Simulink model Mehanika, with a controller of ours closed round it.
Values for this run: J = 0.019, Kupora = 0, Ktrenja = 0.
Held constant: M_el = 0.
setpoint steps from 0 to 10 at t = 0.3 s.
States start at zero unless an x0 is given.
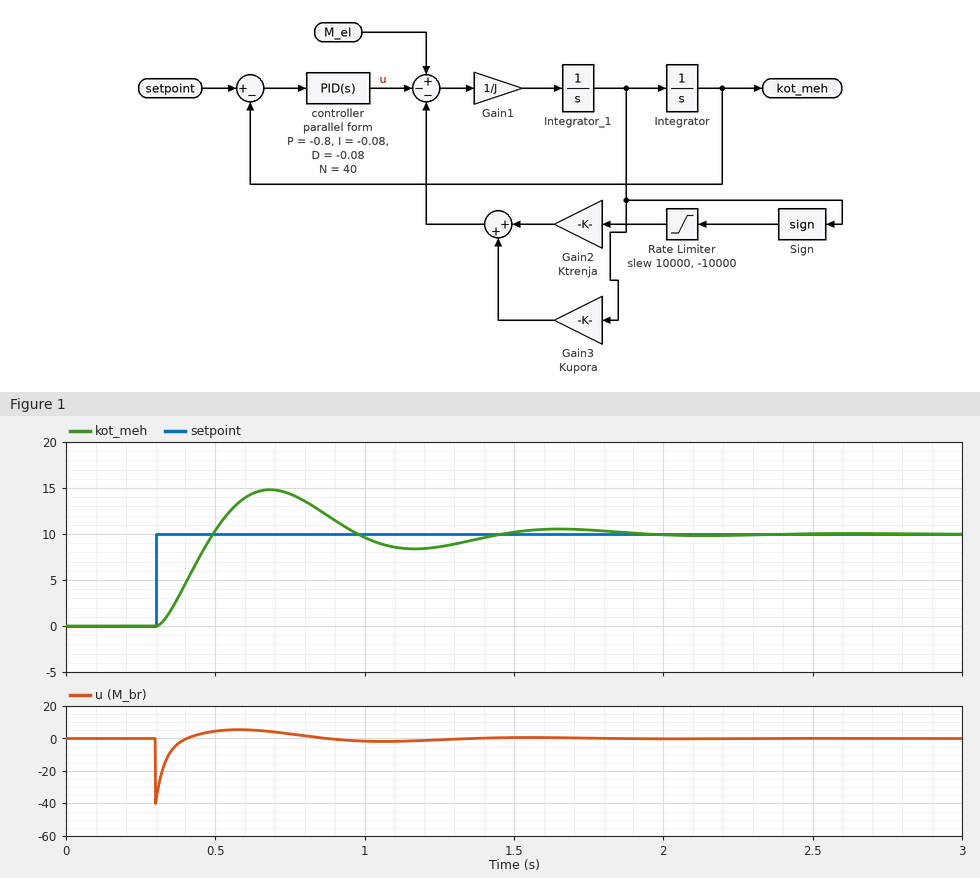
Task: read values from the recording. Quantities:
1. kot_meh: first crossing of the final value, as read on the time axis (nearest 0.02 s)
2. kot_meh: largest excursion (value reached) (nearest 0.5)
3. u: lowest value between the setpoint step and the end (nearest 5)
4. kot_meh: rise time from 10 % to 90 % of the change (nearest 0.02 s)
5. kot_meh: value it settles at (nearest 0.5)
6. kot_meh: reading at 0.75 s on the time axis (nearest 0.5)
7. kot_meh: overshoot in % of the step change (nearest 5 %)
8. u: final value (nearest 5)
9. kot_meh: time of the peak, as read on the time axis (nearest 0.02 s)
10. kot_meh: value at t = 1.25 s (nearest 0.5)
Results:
0.50 s
15.0
-40
0.14 s
10.0
14.5
50 %
0
0.68 s
8.5
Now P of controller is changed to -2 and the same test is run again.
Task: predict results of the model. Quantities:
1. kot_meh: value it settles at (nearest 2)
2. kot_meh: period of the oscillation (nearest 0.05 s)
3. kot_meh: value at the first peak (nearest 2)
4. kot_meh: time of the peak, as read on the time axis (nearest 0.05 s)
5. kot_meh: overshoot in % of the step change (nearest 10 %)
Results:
10
0.60 s
16
0.55 s
60 %
